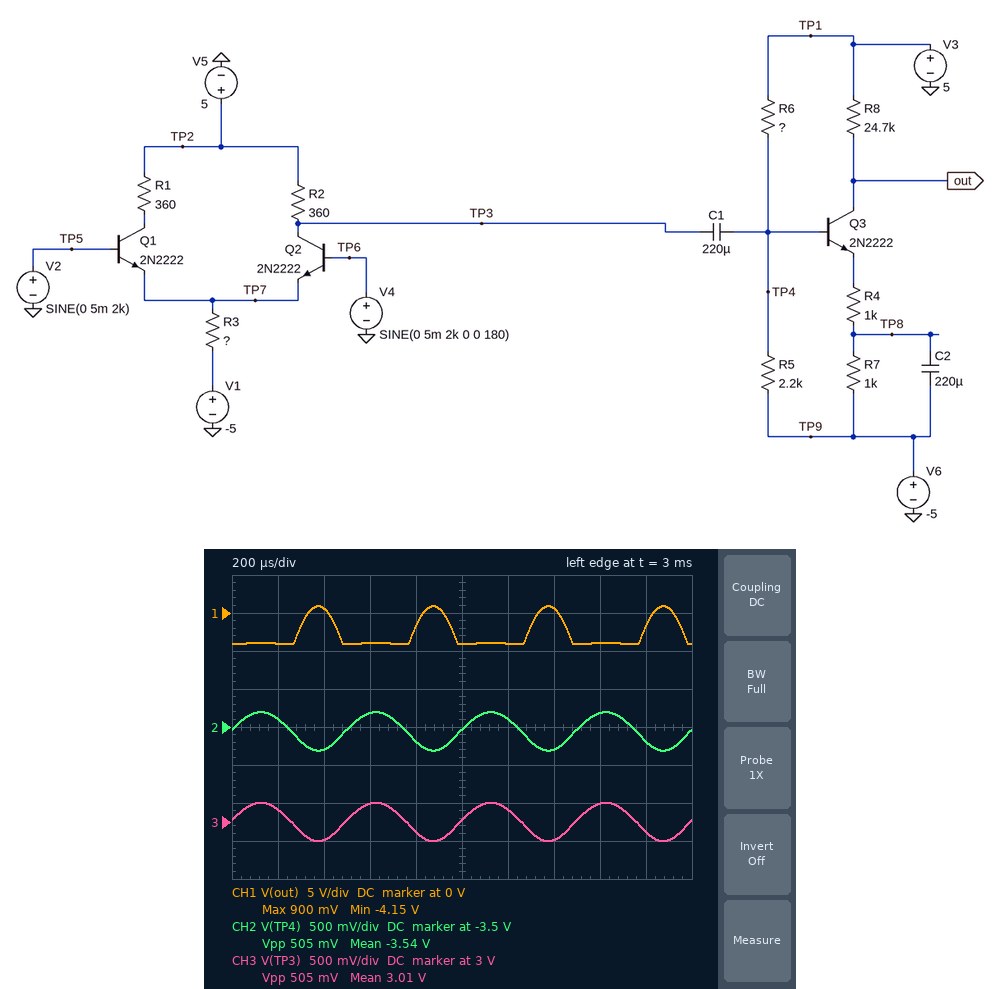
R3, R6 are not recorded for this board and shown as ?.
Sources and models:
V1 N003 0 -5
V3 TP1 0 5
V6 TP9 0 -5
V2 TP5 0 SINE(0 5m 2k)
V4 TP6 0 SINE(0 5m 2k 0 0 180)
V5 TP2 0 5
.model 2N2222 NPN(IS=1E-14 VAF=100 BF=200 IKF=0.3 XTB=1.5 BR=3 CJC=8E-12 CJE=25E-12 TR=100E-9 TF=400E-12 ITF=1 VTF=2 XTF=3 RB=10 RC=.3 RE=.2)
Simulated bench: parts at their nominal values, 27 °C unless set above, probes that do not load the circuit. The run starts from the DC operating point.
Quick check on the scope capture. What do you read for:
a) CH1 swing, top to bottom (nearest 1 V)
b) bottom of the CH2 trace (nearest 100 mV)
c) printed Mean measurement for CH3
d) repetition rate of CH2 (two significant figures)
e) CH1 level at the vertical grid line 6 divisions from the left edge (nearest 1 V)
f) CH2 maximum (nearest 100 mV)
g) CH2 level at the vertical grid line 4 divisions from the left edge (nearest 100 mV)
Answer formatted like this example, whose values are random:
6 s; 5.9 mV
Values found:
5 V; -3.8 V; 3.01 V; 2.0 kHz; -4 V; -3.3 V; -3.7 V
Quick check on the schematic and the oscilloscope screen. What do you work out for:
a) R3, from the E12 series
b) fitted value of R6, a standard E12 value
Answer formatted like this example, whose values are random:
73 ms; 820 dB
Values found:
390 Ω; 12 kΩ
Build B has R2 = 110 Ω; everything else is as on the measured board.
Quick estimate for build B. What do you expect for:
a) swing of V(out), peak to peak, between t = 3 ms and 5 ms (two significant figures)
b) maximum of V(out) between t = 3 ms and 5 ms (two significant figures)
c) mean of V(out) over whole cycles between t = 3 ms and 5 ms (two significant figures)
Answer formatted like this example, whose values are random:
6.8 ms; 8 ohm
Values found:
1.0 V; -3.1 V; -3.9 V
